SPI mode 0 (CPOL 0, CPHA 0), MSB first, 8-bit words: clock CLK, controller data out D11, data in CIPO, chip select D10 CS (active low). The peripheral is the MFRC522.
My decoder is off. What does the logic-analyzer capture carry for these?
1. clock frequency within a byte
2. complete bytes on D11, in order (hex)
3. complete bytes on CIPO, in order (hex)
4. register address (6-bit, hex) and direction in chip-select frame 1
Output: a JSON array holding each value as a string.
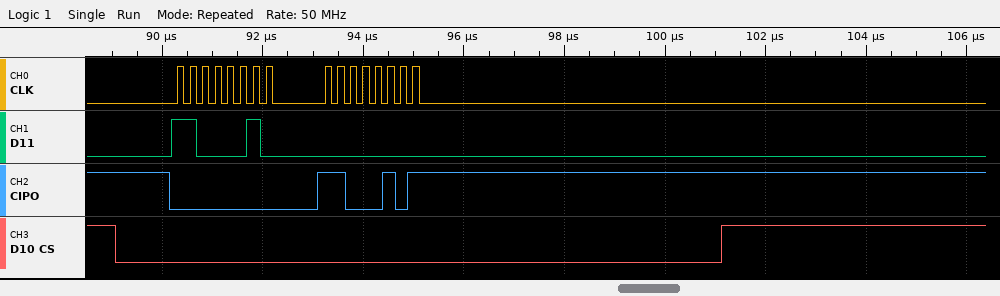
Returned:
["4 MHz", "C2 00", "00 C5", "0x21 read"]
